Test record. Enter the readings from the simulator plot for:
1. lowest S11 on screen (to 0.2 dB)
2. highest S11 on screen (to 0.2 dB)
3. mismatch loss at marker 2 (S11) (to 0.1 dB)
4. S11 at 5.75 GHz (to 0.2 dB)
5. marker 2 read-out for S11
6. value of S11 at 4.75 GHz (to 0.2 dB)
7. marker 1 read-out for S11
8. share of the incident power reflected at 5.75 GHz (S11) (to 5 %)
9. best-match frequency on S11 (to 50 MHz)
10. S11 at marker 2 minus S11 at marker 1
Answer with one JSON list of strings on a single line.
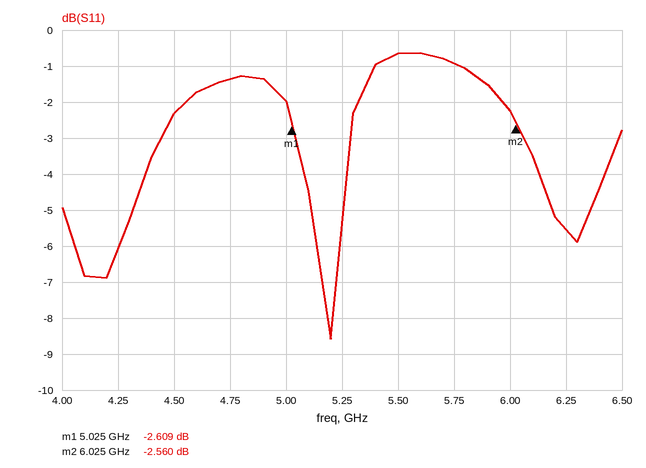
["-8.6 dB", "-0.6 dB", "3.5 dB", "-1.0 dB", "-2.560 dB", "-1.4 dB", "-2.609 dB", "80 %", "5.20 GHz", "0.049 dB"]
